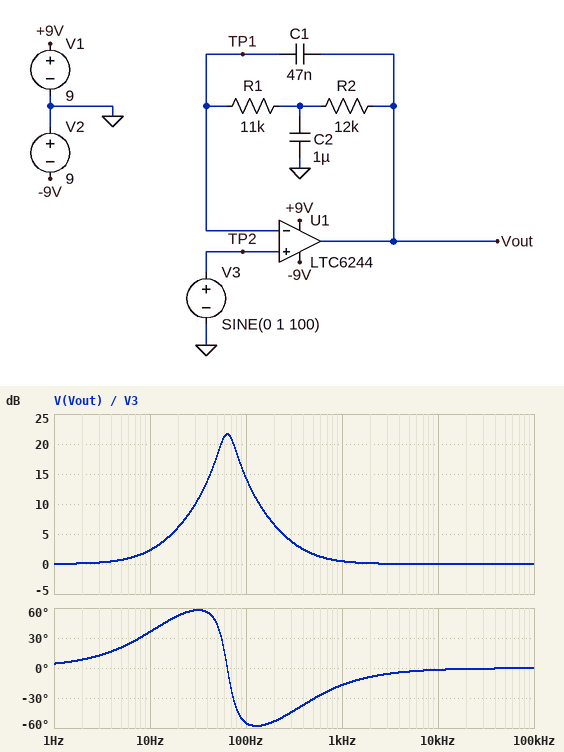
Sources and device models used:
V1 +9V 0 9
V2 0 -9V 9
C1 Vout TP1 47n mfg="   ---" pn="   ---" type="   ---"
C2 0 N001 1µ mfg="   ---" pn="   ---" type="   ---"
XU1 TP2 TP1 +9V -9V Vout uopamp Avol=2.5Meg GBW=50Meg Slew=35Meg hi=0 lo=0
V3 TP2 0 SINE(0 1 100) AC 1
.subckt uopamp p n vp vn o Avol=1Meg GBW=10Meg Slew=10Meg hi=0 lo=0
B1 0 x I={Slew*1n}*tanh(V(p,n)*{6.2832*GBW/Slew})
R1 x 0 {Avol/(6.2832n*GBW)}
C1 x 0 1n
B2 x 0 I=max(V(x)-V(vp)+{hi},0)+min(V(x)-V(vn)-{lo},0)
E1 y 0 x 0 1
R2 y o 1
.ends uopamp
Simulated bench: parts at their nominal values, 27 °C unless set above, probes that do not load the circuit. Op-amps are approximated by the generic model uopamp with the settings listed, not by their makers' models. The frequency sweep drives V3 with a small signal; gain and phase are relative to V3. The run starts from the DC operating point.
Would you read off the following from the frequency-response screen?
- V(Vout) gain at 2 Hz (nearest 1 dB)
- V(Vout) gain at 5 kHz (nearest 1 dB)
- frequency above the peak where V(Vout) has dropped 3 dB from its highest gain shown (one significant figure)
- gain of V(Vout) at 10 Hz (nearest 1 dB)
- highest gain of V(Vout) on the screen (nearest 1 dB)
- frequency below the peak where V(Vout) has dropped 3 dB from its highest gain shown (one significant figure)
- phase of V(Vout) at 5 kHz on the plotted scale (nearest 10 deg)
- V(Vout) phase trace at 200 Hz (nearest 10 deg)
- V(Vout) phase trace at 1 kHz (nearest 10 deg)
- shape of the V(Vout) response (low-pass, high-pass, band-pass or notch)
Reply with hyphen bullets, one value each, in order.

- 0 dB
- 0 dB
- 80 Hz
- 2 dB
- 22 dB
- 50 Hz
- 0 deg
- -50 deg
- -20 deg
- band-pass
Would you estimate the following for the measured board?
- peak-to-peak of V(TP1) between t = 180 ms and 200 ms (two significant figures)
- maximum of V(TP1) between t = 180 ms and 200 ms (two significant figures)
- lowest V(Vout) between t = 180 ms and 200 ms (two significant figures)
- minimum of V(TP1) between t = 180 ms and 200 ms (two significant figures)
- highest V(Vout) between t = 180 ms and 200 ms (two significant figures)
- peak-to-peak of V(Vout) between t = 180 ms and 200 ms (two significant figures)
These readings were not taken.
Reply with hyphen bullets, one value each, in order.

- 2.0 V
- 1.0 V
- -5.2 V
- -1.0 V
- 5.2 V
- 10 V
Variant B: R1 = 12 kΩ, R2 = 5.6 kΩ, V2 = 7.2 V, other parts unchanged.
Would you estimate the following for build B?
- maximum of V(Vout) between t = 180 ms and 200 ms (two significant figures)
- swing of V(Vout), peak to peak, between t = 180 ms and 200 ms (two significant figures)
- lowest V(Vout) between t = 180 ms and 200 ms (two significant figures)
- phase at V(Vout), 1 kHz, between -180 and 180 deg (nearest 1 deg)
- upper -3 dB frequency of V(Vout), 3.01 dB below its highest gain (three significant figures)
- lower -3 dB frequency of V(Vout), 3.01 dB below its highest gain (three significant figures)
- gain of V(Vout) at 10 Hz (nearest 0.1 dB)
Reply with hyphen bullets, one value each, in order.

- 7.0 V
- 14 V
- -7.0 V
- -16 deg
- 113 Hz
- 70.8 Hz
- 0.7 dB
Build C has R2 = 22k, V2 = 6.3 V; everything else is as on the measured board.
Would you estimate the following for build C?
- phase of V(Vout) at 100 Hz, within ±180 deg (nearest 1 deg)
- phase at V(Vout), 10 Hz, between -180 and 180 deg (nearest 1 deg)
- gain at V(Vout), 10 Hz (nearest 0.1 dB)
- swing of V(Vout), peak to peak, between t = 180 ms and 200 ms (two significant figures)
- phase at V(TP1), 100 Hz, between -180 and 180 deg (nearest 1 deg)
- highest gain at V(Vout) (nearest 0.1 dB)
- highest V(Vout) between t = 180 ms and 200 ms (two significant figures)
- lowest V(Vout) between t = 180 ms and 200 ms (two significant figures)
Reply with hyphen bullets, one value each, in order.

- -61 deg
- 51 deg
- 5.3 dB
- 8.4 V
- 0 deg
- 23.6 dB
- 4.2 V
- -4.2 V
